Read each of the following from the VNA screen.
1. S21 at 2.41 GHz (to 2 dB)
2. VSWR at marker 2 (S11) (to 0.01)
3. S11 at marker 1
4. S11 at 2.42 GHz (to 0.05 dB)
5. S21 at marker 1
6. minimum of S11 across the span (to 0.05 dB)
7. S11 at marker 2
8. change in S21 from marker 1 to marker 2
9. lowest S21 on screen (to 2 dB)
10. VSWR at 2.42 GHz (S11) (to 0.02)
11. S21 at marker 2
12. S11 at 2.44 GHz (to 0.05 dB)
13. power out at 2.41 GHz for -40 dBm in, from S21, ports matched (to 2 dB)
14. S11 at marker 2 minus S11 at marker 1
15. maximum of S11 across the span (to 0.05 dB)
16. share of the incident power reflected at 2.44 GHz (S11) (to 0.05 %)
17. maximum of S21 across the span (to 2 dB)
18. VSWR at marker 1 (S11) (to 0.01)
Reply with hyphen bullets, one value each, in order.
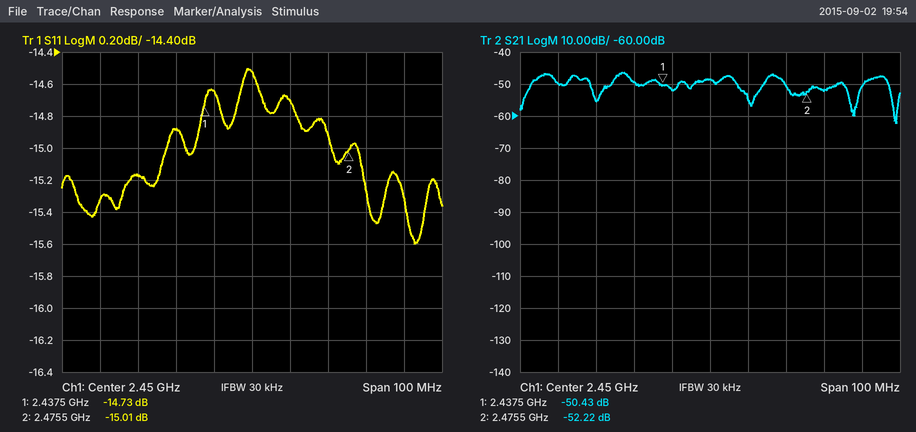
- -50 dB
- 1.43
- -14.73 dB
- -15.15 dB
- -50.43 dB
- -15.60 dB
- -15.01 dB
- -1.79 dB
- -62 dB
- 1.42
- -52.22 dB
- -14.65 dB
- -90 dBm
- -0.28 dB
- -14.50 dB
- 3.45 %
- -46 dB
- 1.45
